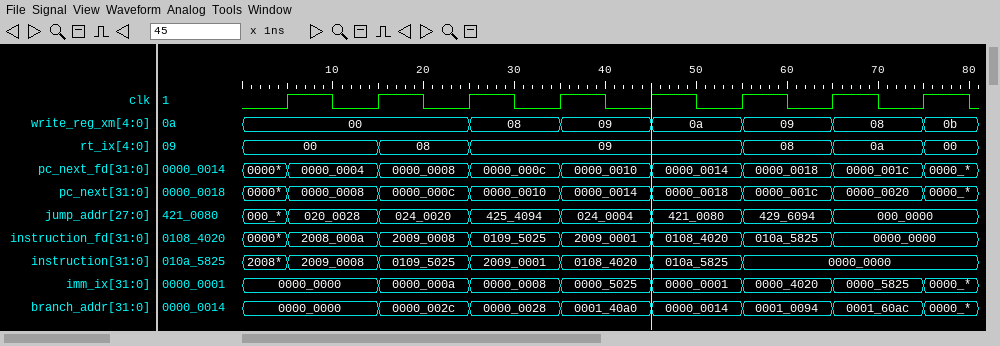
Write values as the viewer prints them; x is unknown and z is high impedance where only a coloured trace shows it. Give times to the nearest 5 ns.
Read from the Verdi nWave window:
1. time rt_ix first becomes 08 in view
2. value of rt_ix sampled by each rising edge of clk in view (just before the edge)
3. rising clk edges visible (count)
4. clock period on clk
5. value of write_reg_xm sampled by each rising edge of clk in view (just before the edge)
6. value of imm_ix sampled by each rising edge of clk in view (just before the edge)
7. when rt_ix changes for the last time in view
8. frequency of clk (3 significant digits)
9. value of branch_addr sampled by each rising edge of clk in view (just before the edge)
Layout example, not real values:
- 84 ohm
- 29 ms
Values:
- 15 ns
- 00, 00, 08, 09, 09, 09, 08, 0a
- 8
- 10 ns
- 00, 00, 00, 08, 09, 0a, 09, 08
- 0000_0000, 0000_0000, 0000_000a, 0000_0008, 0000_5025, 0000_0001, 0000_4020, 0000_5825
- 75 ns
- 100 MHz
- 0000_0000, 0000_0000, 0000_002c, 0000_0028, 0001_40a0, 0000_0014, 0001_0094, 0001_60ac
